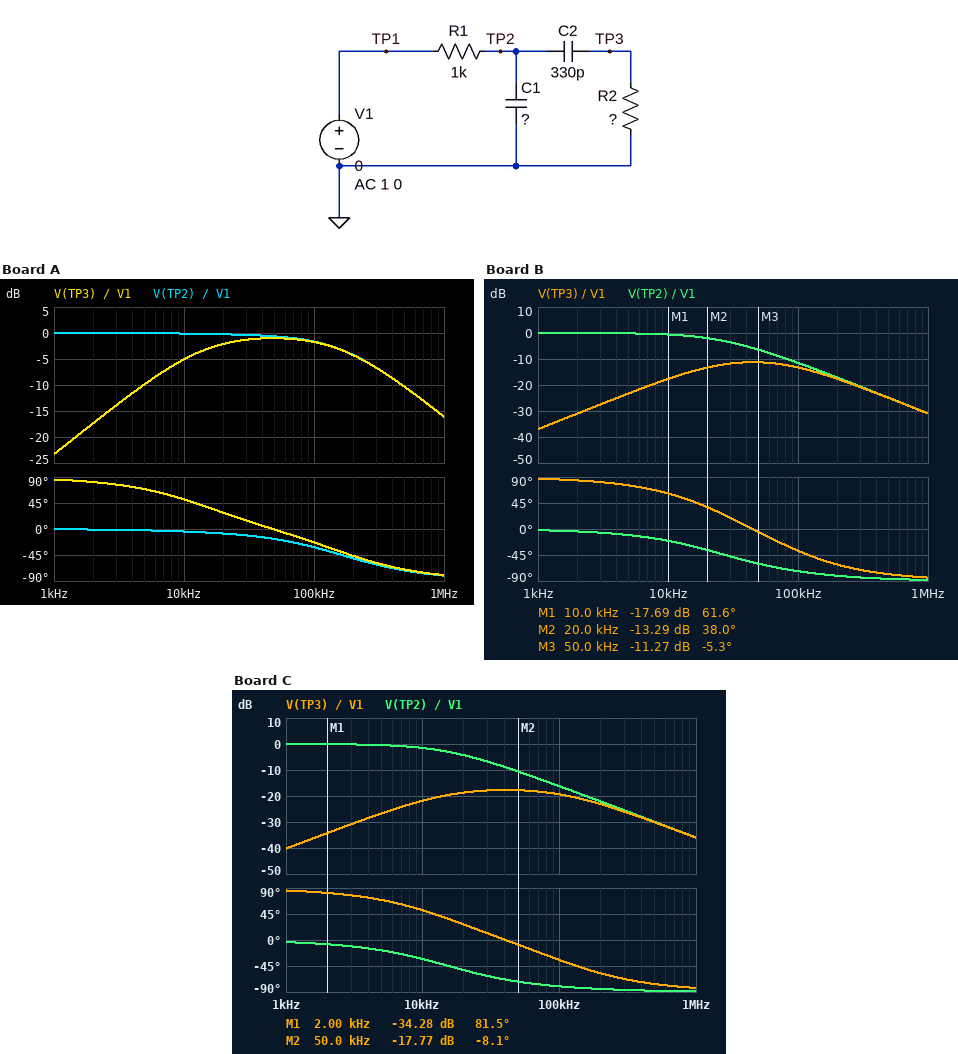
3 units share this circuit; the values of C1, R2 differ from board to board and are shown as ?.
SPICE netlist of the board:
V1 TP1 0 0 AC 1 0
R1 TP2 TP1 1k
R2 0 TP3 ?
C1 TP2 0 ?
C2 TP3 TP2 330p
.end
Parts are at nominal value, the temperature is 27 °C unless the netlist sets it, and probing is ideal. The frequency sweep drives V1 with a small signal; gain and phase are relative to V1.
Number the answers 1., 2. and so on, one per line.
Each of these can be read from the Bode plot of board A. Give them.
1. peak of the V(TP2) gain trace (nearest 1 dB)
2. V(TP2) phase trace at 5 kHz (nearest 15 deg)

1. 0 dB
2. 0 deg
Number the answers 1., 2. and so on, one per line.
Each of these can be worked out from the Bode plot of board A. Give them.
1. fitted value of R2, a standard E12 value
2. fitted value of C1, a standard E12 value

1. 33 kΩ
2. 1 nF
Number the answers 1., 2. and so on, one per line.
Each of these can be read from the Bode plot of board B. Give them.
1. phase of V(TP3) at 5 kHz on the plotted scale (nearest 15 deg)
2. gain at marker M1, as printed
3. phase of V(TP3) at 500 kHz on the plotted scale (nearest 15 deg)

1. 75 deg
2. -17.69 dB
3. -75 deg
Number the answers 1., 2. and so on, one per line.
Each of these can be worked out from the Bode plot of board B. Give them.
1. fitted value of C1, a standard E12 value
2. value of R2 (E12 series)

1. 5.6 nF
2. 6.8 kΩ
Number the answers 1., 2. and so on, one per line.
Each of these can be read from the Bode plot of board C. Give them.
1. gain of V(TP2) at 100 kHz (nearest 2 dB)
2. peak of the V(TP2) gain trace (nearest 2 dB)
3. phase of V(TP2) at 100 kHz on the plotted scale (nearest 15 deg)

1. -16 dB
2. 0 dB
3. -75 deg
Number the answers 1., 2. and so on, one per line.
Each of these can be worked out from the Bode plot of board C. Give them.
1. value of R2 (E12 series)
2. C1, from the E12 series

1. 4.7 kΩ
2. 10 nF
